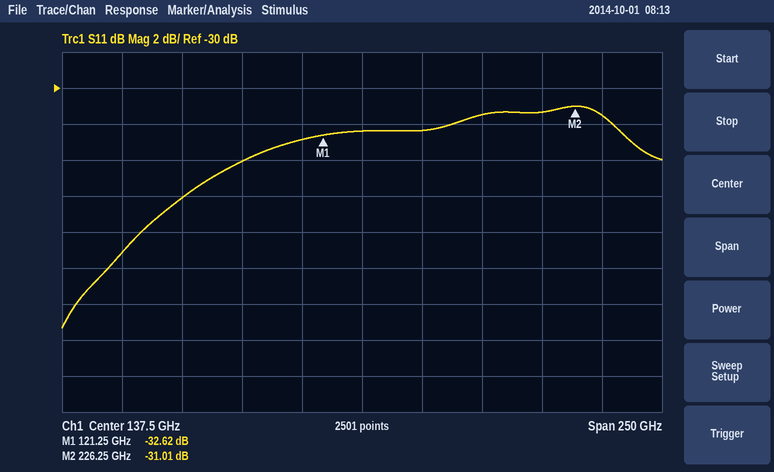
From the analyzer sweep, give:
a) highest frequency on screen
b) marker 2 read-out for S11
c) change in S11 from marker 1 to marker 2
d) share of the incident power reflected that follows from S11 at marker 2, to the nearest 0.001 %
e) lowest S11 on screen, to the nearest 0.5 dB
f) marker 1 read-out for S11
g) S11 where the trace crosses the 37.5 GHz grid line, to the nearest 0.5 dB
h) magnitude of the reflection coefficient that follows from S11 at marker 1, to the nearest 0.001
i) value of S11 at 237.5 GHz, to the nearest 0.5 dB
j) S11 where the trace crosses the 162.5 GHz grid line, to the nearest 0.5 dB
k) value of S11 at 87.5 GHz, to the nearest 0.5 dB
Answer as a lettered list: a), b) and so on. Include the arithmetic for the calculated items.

a) 262.5 GHz
b) -31.01 dB
c) -31.01 − (-32.62) = 1.61 dB
d) 10^(-31.01/10) ≈ 0.079 %
e) -43.5 dB
f) -32.62 dB
g) -39.0 dB
h) 10^(-32.62/20) ≈ 0.023
i) -31.5 dB
j) -32.5 dB
k) -34.0 dB
